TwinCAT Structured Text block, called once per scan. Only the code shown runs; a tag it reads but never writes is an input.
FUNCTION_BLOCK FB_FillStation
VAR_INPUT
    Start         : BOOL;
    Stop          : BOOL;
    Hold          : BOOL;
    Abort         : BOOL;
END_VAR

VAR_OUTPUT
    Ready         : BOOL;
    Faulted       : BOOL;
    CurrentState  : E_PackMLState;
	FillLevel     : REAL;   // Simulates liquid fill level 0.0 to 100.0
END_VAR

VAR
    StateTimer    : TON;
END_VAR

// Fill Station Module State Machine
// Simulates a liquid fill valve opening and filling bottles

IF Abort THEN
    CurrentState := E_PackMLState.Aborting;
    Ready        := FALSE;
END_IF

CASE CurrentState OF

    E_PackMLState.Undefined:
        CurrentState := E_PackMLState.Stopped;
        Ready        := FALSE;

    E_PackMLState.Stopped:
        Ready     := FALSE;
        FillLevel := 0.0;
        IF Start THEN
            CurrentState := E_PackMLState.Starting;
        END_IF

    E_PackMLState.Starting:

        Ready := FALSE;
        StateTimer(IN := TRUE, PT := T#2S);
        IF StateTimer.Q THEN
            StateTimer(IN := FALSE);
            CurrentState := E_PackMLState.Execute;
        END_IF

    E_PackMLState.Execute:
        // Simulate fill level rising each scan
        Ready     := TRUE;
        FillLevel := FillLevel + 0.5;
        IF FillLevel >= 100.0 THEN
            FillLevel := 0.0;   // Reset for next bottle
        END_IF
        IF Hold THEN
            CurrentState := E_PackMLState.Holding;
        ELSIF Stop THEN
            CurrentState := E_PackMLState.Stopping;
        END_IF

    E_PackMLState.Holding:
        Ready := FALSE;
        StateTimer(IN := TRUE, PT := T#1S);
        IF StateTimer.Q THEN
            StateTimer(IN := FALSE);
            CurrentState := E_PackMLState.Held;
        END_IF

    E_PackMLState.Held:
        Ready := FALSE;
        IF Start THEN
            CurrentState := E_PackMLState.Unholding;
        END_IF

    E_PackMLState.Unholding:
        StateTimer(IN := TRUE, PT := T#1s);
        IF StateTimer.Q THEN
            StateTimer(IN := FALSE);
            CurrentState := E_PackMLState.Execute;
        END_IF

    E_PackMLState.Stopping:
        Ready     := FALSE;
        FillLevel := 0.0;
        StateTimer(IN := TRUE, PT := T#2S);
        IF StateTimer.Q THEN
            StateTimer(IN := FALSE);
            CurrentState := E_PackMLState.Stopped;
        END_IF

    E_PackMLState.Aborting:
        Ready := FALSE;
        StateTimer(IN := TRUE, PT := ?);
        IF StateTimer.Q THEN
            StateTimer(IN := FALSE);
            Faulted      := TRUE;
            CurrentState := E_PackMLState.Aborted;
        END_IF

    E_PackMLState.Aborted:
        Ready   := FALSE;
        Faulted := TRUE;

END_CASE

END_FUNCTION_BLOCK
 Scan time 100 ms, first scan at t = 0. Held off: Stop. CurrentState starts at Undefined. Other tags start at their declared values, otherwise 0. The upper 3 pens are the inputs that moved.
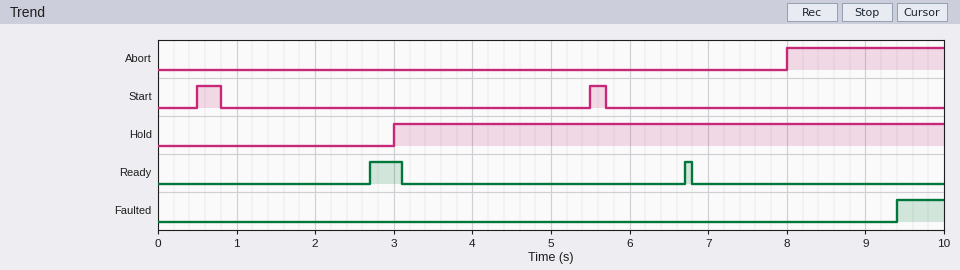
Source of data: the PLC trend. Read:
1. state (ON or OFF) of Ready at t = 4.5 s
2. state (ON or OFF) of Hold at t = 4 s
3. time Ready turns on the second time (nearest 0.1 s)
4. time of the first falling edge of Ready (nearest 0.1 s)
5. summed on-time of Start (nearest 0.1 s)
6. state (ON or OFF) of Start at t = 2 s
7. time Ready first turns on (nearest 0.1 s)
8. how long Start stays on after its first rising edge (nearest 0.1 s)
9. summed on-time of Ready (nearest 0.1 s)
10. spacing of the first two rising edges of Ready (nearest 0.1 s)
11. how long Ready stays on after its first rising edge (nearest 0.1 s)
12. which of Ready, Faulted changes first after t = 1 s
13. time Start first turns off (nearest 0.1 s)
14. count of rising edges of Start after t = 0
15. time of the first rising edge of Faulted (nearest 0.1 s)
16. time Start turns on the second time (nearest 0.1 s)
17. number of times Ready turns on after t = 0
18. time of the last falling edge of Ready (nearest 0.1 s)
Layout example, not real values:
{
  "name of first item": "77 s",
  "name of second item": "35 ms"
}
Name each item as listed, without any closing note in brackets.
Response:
{
  "state (ON or OFF) of Ready at t = 4.5 s": "OFF",
  "state (ON or OFF) of Hold at t = 4 s": "ON",
  "time Ready turns on the second time": "6.7 s",
  "time of the first falling edge of Ready": "3.1 s",
  "summed on-time of Start": "0.5 s",
  "state (ON or OFF) of Start at t = 2 s": "OFF",
  "time Ready first turns on": "2.7 s",
  "how long Start stays on after its first rising edge": "0.3 s",
  "summed on-time of Ready": "0.5 s",
  "spacing of the first two rising edges of Ready": "4.0 s",
  "how long Ready stays on after its first rising edge": "0.4 s",
  "which of Ready, Faulted changes first after t = 1 s": "Ready",
  "time Start first turns off": "0.8 s",
  "count of rising edges of Start after t = 0": "2",
  "time of the first rising edge of Faulted": "9.4 s",
  "time Start turns on the second time": "5.5 s",
  "number of times Ready turns on after t = 0": "2",
  "time of the last falling edge of Ready": "6.8 s"
}
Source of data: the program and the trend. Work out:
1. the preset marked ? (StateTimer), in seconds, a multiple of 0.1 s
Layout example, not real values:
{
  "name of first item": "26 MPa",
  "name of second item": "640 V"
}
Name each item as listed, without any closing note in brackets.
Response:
{
  "the preset marked ? (StateTimer), in seconds, a multiple of 0.1 s": "1.4 s"
}
